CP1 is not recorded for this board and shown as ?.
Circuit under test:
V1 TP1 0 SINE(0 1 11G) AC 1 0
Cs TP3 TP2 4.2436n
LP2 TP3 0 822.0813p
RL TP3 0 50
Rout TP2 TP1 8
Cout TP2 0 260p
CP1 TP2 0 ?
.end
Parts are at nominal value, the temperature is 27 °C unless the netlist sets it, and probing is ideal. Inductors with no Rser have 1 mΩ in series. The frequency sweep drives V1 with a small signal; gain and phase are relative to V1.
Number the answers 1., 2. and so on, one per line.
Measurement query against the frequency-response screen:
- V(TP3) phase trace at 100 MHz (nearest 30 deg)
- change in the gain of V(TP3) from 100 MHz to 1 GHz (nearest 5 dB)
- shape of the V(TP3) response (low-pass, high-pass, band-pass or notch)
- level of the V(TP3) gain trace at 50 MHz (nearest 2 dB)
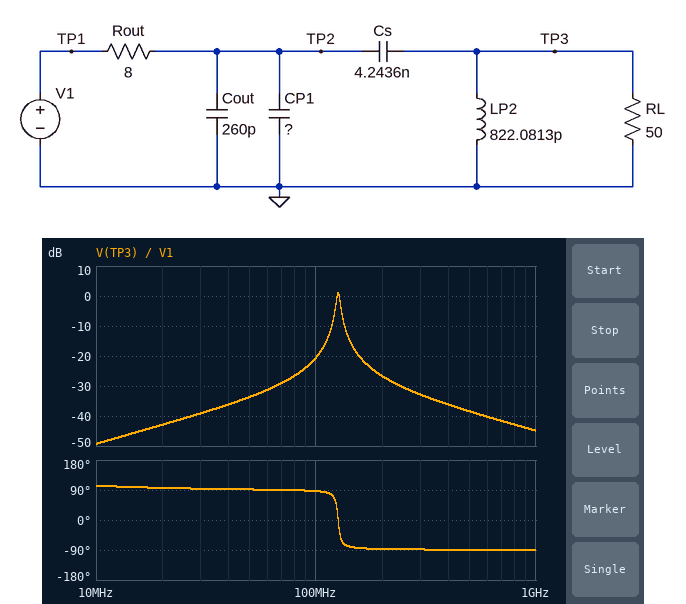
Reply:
1. 90 deg
2. -25 dB
3. band-pass
4. -34 dB
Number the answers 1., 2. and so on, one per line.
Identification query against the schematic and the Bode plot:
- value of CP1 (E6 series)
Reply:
1. 3.3 nF
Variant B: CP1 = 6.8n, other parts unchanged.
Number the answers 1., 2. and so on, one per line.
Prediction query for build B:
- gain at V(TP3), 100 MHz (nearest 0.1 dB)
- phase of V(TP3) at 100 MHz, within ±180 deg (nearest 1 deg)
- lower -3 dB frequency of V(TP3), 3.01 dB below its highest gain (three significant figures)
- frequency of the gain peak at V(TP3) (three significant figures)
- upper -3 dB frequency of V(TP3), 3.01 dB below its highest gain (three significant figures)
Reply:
1. -15.3 dB
2. 82 deg
3. 107 MHz
4. 108 MHz
5. 109 MHz
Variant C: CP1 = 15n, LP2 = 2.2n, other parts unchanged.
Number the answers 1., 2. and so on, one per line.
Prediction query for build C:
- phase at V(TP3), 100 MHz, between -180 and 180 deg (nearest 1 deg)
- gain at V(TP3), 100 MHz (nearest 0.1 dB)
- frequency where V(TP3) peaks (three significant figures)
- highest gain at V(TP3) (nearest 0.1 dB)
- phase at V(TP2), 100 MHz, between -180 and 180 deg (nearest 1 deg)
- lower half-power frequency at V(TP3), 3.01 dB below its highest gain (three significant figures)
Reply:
1. -88 deg
2. -34.0 dB
3. 58.9 MHz
4. -0.1 dB
5. -89 deg
6. 58.2 MHz
